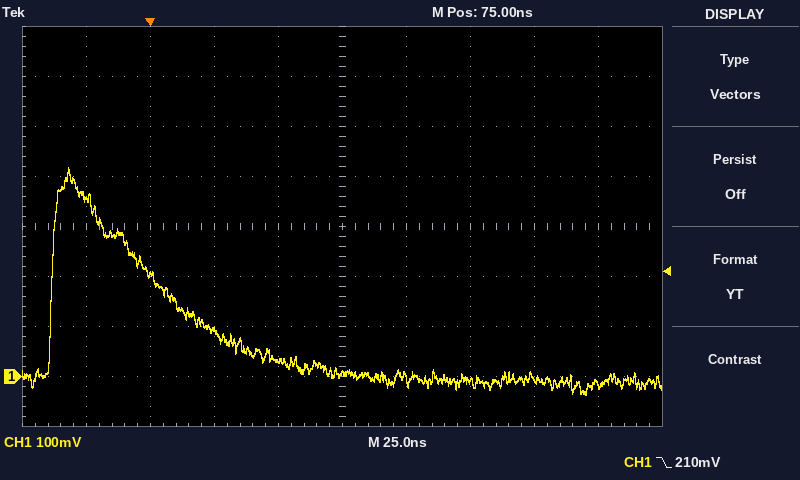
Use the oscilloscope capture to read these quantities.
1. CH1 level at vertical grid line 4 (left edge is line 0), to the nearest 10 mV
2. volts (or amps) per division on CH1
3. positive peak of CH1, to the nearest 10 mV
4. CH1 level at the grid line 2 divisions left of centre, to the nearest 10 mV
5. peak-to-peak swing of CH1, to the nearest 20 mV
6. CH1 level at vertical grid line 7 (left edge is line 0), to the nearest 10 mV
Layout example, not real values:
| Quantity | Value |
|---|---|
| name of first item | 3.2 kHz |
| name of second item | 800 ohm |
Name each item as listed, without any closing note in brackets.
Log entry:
| Quantity | Value |
|---|---|
| CH1 level at vertical grid line 4 (left edge is line 0), to the nearest 10 mV | 30 mV |
| volts (or amps) per division on CH1 | 100 mV |
| positive peak of CH1, to the nearest 10 mV | 420 mV |
| CH1 level at the grid line 2 divisions left of centre, to the nearest 10 mV | 90 mV |
| peak-to-peak swing of CH1, to the nearest 20 mV | 460 mV |
| CH1 level at vertical grid line 7 (left edge is line 0), to the nearest 10 mV | -10 mV |
